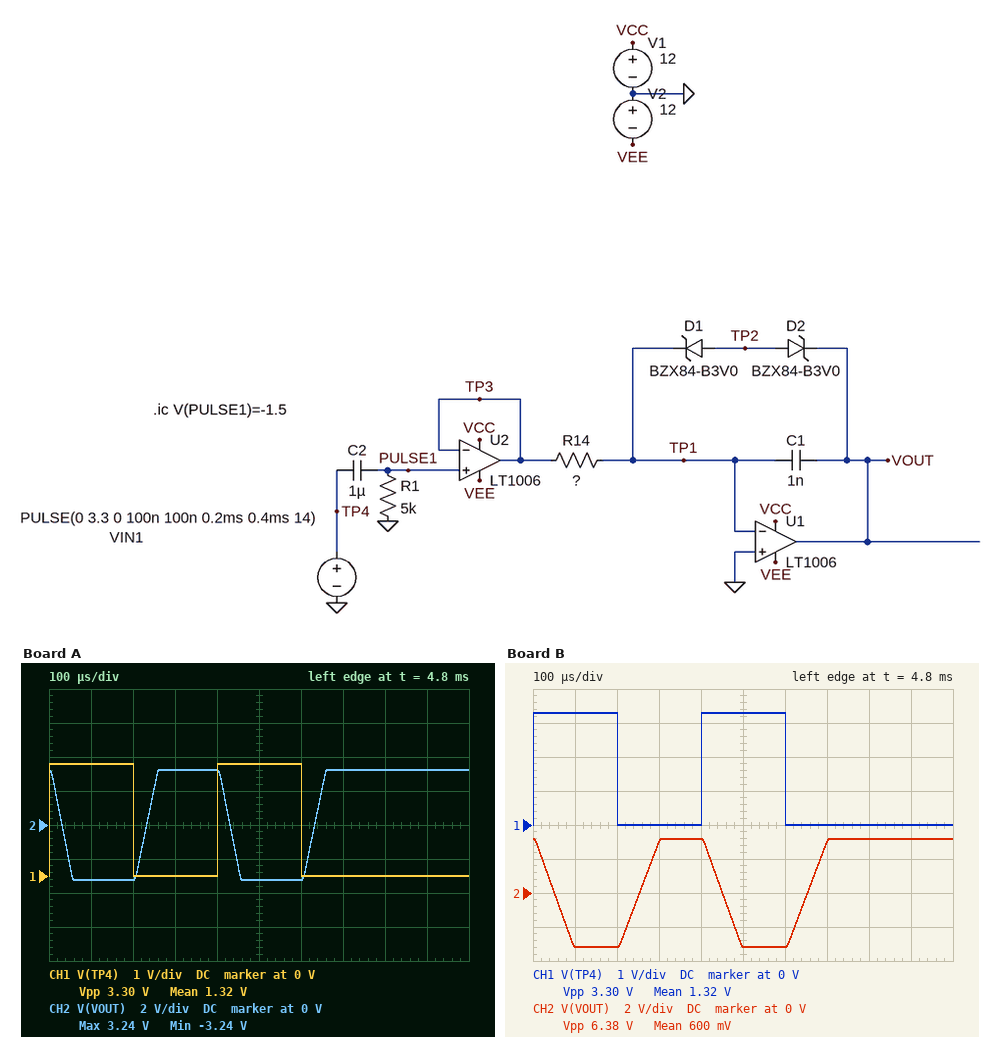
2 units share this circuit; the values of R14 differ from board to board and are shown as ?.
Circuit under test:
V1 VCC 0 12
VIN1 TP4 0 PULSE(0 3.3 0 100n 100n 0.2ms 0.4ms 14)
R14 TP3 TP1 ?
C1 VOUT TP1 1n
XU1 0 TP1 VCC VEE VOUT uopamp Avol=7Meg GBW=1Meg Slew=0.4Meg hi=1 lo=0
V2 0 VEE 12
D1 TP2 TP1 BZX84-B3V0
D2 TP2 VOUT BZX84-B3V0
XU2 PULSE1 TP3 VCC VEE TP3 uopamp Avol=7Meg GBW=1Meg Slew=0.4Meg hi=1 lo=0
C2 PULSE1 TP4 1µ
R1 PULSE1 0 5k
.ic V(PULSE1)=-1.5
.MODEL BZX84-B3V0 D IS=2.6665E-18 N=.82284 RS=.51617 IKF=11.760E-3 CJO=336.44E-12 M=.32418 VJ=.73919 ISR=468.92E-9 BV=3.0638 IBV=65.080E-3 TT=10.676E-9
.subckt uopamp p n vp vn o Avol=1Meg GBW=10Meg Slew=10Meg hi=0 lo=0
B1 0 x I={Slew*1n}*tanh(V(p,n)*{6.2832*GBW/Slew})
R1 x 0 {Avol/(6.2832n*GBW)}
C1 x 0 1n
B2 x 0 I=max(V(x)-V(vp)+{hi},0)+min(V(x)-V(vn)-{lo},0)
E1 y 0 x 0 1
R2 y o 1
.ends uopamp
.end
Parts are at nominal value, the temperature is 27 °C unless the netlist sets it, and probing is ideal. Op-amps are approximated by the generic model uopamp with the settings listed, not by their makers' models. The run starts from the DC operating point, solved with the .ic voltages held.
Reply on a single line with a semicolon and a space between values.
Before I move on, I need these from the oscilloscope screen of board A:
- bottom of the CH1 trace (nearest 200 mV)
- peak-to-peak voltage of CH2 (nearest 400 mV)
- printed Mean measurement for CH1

0 V; 6.4 V; 1.32 V
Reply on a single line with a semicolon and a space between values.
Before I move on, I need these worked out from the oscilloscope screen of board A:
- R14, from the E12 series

12 kΩ
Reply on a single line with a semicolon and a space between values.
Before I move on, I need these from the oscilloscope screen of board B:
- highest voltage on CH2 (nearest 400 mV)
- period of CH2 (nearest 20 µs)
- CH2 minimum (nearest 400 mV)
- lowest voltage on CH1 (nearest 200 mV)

3.2 V; 400 µs; -3.2 V; 0 V
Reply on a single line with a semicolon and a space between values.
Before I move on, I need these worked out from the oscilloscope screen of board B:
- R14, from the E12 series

22 kΩ
